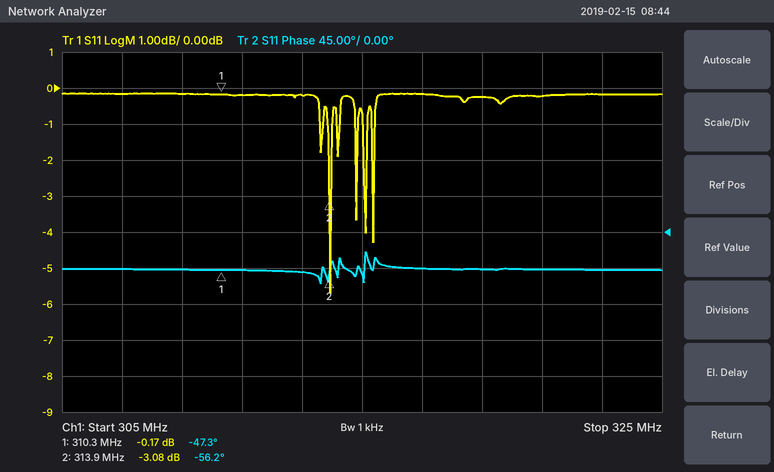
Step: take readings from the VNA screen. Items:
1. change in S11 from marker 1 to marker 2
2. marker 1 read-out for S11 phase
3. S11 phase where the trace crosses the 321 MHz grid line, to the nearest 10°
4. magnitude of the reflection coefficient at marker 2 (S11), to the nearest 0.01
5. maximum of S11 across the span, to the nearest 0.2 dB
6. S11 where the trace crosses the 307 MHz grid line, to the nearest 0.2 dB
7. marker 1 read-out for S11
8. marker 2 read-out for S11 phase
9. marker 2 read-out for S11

-2.91 dB
-47.3°
-50°
0.70
-0.2 dB
-0.2 dB
-0.17 dB
-56.2°
-3.08 dB
